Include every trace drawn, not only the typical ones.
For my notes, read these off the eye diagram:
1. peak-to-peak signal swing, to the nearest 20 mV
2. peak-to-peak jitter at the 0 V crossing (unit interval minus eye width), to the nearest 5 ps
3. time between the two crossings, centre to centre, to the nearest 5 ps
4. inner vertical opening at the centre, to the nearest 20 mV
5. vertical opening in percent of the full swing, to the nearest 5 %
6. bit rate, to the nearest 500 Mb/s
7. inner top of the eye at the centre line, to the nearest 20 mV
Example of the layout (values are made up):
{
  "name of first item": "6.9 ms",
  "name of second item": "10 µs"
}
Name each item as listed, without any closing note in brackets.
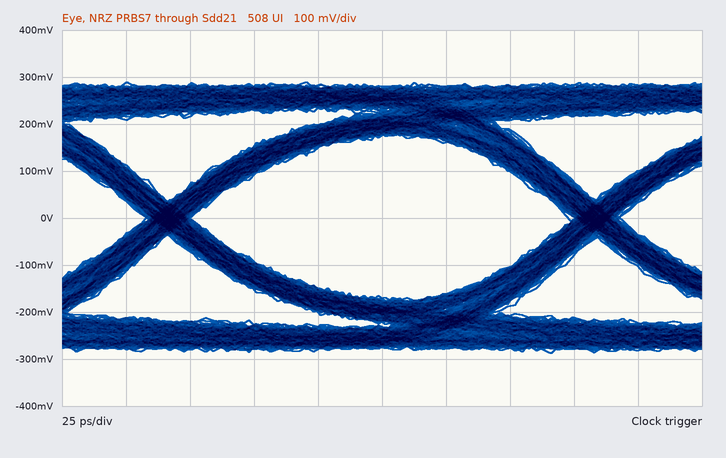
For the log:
{
  "peak-to-peak signal swing, to the nearest 20 mV": "580 mV",
  "peak-to-peak jitter at the 0 V crossing (unit interval minus eye width), to the nearest 5 ps": "20 ps",
  "time between the two crossings, centre to centre, to the nearest 5 ps": "165 ps",
  "inner vertical opening at the centre, to the nearest 20 mV": "340 mV",
  "vertical opening in percent of the full swing, to the nearest 5 %": "60 %",
  "bit rate, to the nearest 500 Mb/s": "6.0 Gb/s",
  "inner top of the eye at the centre line, to the nearest 20 mV": "180 mV"
}
